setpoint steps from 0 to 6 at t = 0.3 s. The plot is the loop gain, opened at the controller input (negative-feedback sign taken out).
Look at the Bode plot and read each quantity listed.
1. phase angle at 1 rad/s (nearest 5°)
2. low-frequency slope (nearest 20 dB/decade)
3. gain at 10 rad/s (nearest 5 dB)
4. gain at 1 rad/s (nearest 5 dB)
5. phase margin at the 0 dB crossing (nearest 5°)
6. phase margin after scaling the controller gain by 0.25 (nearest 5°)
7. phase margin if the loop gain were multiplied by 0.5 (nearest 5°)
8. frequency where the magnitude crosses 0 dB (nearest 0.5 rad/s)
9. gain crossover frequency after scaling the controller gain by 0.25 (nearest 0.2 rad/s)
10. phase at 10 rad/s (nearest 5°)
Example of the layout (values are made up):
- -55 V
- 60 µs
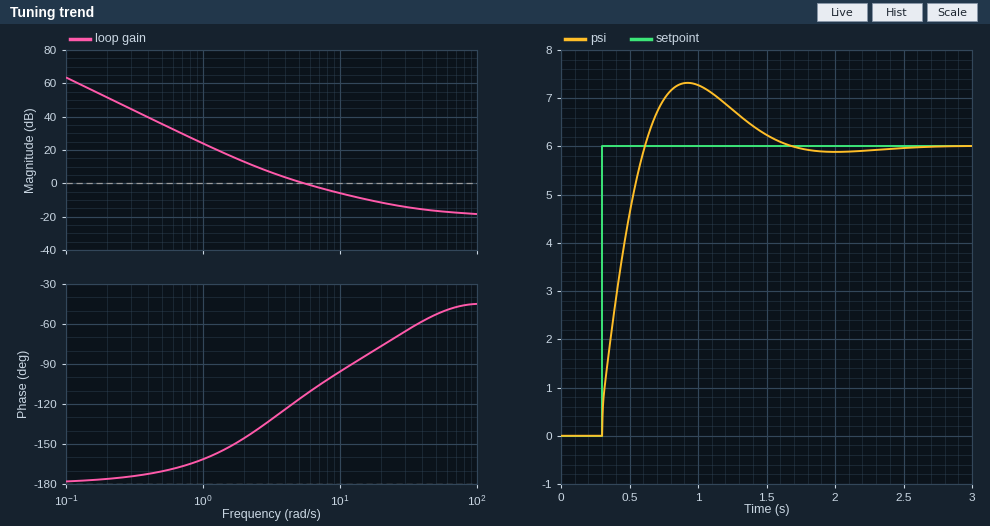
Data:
- -160°
- -40 dB/decade
- -5 dB
- 25 dB
- 65°
- 35°
- 50°
- 5.5 rad/s
- 2.2 rad/s
- -95°
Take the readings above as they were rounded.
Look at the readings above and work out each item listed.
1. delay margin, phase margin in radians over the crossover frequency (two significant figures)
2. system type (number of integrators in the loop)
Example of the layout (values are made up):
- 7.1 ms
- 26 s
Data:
- 0.21 s
- 2
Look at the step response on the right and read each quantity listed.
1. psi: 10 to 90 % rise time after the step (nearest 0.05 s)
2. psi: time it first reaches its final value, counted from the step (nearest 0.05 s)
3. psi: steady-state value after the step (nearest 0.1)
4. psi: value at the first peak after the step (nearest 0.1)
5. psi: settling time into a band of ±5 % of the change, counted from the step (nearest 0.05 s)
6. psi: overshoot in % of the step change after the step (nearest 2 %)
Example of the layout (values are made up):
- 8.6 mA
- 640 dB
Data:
- 0.25 s
- 0.30 s
- 6.0
- 7.3
- 1.15 s
- 22 %
